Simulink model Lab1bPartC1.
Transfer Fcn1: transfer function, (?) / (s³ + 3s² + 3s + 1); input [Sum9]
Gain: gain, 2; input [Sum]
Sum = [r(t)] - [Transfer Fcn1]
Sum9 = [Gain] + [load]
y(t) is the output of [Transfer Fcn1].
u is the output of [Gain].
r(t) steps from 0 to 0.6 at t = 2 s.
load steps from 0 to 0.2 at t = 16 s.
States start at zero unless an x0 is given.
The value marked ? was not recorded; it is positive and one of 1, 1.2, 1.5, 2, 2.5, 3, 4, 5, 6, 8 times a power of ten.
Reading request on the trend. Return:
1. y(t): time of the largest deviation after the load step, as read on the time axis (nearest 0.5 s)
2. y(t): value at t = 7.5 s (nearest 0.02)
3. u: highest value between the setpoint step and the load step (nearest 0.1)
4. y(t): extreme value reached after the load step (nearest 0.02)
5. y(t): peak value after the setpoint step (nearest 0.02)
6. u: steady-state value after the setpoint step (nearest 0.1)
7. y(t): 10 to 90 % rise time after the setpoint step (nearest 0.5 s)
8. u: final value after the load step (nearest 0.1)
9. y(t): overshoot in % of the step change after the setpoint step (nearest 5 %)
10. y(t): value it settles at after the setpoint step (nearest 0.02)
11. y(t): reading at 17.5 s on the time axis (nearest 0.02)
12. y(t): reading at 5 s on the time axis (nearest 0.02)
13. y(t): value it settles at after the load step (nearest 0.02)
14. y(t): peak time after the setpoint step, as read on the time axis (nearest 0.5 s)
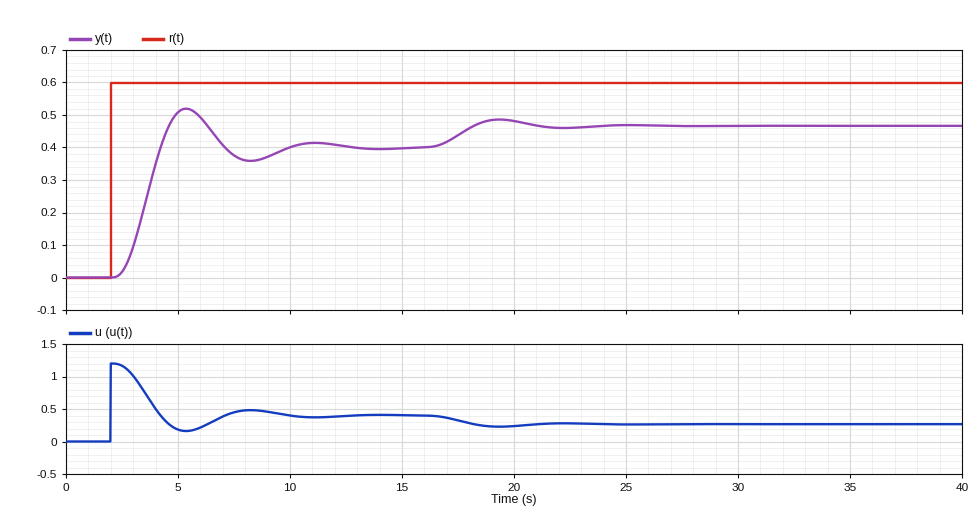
19.5 s
0.38
1.2
0.48
0.52
0.4
1.5 s
0.3
30 %
0.40
0.44
0.50
0.46
5.5 s
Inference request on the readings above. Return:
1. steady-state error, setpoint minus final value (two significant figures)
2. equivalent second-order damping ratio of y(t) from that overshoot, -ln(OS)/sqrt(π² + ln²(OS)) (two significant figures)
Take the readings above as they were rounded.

0.20
0.36
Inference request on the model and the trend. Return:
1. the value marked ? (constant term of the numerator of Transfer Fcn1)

1
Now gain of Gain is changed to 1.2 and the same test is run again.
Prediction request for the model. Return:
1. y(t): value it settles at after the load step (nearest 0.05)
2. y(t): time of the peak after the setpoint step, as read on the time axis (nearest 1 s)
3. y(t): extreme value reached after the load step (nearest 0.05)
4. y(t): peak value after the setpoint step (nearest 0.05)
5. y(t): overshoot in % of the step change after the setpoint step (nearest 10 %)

0.40
6 s
0.45
0.40
20 %
